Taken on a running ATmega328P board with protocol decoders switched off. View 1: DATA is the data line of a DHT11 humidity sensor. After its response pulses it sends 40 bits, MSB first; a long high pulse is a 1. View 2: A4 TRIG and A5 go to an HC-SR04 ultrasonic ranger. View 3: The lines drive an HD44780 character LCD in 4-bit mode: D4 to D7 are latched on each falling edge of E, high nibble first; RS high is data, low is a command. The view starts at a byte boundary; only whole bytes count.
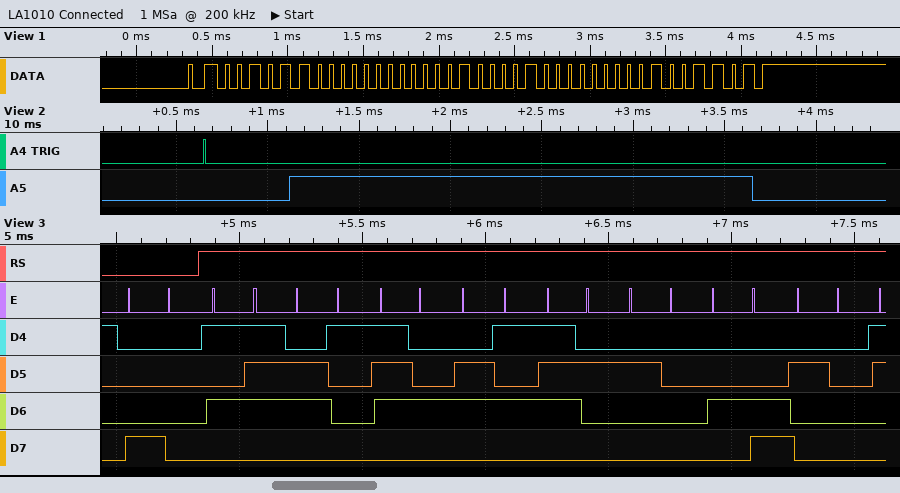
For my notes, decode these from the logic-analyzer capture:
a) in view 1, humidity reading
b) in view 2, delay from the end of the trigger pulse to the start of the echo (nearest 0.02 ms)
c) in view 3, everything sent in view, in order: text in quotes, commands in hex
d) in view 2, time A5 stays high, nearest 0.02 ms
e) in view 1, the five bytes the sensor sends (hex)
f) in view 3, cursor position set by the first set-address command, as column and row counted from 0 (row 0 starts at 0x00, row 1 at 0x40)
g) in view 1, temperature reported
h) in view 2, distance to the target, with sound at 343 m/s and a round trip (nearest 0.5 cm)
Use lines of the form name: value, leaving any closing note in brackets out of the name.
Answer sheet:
in view 1, humidity reading: 44 %
in view 2, delay from the end of the trigger pulse to the start of the echo: 0.46 ms
in view 3, everything sent in view, in order: text in quotes, commands in hex: 0x80 "Water L "
in view 2, time A5 stays high, nearest 0.02 ms: 2.54 ms
in view 1, the five bytes the sensor sends: 2C 00 21 00 4D
in view 3, cursor position set by the first set-address command, as column and row counted from 0: column 0, row 0
in view 1, temperature reported: 33.0 °C
in view 2, distance to the target, with sound at 343 m/s and a round trip: 43.5 cm
